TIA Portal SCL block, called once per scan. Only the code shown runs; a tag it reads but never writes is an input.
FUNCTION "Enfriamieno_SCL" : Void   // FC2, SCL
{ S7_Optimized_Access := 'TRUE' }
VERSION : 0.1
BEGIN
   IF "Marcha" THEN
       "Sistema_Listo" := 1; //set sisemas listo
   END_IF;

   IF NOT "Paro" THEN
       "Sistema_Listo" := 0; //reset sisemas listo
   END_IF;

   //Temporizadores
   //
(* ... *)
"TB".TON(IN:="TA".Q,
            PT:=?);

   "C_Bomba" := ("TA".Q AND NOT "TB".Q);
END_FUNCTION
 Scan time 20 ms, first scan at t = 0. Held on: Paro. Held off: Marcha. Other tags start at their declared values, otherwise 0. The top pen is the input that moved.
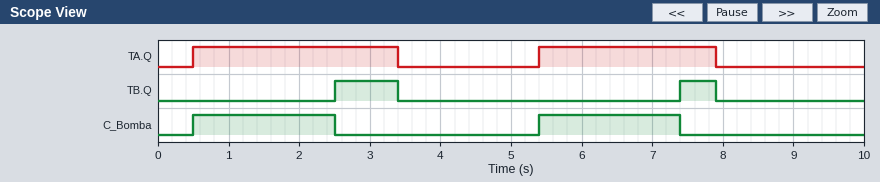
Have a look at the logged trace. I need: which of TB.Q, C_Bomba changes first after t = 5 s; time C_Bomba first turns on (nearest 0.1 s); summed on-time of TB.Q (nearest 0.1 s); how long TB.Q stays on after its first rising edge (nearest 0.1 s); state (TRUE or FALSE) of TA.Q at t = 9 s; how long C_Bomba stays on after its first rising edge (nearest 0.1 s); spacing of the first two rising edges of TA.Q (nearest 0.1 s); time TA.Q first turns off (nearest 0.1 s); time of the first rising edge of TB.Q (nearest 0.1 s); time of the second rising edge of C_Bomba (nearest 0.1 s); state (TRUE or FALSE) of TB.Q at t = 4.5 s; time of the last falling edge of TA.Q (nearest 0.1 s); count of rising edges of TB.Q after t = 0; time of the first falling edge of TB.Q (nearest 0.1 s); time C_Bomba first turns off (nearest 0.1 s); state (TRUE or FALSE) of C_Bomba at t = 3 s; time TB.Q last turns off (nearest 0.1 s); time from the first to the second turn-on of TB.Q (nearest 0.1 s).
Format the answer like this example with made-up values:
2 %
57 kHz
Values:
C_Bomba
0.5 s
1.4 s
0.9 s
FALSE
2.0 s
4.9 s
3.4 s
2.5 s
5.4 s
FALSE
7.9 s
2
3.4 s
2.5 s
FALSE
7.9 s
4.9 s
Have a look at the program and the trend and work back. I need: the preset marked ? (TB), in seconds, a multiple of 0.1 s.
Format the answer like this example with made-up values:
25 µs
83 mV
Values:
2.0 s
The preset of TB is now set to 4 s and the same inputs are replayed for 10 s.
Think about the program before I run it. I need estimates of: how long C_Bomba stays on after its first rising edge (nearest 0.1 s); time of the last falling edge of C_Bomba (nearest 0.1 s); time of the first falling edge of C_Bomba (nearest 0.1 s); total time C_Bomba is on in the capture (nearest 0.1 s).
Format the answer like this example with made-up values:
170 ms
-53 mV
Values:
2.9 s
7.9 s
3.4 s
5.4 s
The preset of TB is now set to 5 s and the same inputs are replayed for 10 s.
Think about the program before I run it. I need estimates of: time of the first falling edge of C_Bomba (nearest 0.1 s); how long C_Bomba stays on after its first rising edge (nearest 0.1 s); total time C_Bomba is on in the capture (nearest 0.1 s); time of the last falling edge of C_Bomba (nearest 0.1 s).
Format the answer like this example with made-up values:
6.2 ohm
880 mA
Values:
3.4 s
2.9 s
5.4 s
7.9 s
